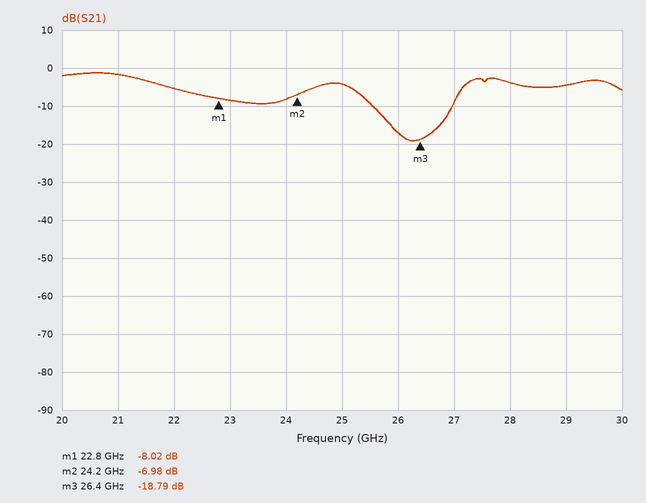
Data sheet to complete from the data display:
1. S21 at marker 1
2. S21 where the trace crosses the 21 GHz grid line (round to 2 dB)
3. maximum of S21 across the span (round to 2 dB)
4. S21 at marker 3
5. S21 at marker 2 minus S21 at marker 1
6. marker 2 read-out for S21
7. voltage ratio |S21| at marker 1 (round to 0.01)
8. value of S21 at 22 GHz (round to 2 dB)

-8.02 dB
-2 dB
-2 dB
-18.79 dB
1.04 dB
-6.98 dB
0.40
-6 dB
